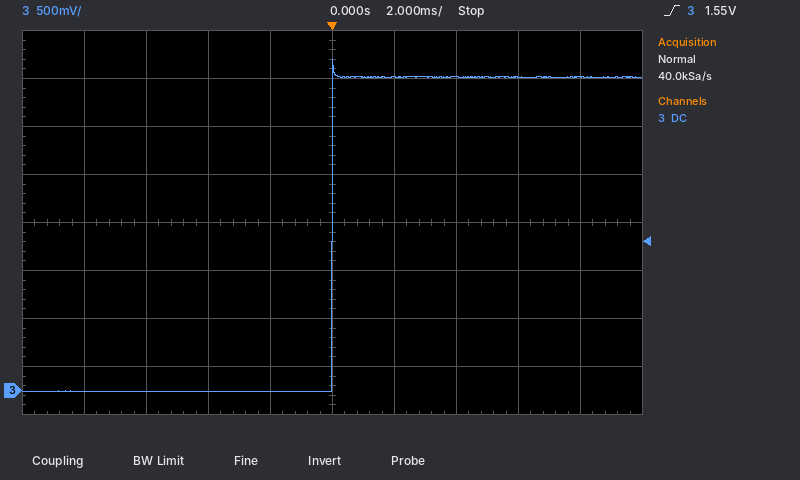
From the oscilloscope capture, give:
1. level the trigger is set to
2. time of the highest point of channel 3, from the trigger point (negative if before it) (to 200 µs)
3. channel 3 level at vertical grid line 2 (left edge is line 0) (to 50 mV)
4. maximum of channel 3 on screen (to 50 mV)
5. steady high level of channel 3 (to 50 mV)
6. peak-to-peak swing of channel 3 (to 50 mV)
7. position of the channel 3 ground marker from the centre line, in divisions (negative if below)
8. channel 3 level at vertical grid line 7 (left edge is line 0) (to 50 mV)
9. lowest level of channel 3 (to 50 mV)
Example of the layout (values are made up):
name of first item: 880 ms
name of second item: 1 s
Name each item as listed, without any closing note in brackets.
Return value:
level the trigger is set to: 1.55 V
time of the highest point of channel 3, from the trigger point (negative if before it): 0.0 ms
channel 3 level at vertical grid line 2 (left edge is line 0): 0 mV
maximum of channel 3 on screen: 3.45 V
steady high level of channel 3: 3.25 V
peak-to-peak swing of channel 3: 3.45 V
position of the channel 3 ground marker from the centre line, in divisions: -3.5 div
channel 3 level at vertical grid line 7 (left edge is line 0): 3.25 V
lowest level of channel 3: 0 mV
